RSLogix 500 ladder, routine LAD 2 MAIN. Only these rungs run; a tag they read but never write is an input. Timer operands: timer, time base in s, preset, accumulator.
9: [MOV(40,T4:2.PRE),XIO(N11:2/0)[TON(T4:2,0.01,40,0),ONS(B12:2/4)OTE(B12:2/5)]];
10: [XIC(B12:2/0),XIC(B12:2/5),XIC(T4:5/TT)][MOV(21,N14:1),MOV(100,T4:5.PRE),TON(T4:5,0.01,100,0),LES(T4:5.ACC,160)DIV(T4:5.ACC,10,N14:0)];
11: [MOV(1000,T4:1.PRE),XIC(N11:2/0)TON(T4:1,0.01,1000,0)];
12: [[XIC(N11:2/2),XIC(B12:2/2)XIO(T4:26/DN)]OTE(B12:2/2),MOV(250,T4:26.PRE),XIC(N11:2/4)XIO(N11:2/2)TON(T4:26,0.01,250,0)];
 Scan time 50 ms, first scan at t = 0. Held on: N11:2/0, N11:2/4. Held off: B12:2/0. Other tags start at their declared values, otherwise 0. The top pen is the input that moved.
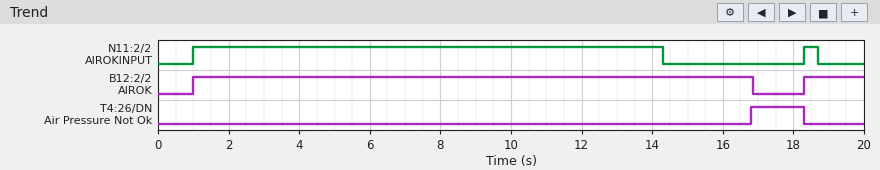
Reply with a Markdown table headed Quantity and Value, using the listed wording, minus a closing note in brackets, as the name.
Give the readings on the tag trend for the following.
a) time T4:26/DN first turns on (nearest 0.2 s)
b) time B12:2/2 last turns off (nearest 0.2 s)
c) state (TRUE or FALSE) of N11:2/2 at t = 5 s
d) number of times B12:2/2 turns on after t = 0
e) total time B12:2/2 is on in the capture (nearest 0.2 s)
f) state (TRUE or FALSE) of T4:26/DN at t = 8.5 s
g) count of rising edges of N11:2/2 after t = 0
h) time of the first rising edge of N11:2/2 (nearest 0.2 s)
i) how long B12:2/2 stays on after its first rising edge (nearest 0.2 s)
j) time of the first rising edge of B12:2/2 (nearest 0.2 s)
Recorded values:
| Quantity | Value |
|---|---|
| time T4:26/DN first turns on | 16.8 s |
| time B12:2/2 last turns off | 16.8 s |
| state (TRUE or FALSE) of N11:2/2 at t = 5 s | TRUE |
| number of times B12:2/2 turns on after t = 0 | 2 |
| total time B12:2/2 is on in the capture | 17.6 s |
| state (TRUE or FALSE) of T4:26/DN at t = 8.5 s | FALSE |
| count of rising edges of N11:2/2 after t = 0 | 2 |
| time of the first rising edge of N11:2/2 | 1.0 s |
| how long B12:2/2 stays on after its first rising edge | 15.8 s |
| time of the first rising edge of B12:2/2 | 1.0 s |
